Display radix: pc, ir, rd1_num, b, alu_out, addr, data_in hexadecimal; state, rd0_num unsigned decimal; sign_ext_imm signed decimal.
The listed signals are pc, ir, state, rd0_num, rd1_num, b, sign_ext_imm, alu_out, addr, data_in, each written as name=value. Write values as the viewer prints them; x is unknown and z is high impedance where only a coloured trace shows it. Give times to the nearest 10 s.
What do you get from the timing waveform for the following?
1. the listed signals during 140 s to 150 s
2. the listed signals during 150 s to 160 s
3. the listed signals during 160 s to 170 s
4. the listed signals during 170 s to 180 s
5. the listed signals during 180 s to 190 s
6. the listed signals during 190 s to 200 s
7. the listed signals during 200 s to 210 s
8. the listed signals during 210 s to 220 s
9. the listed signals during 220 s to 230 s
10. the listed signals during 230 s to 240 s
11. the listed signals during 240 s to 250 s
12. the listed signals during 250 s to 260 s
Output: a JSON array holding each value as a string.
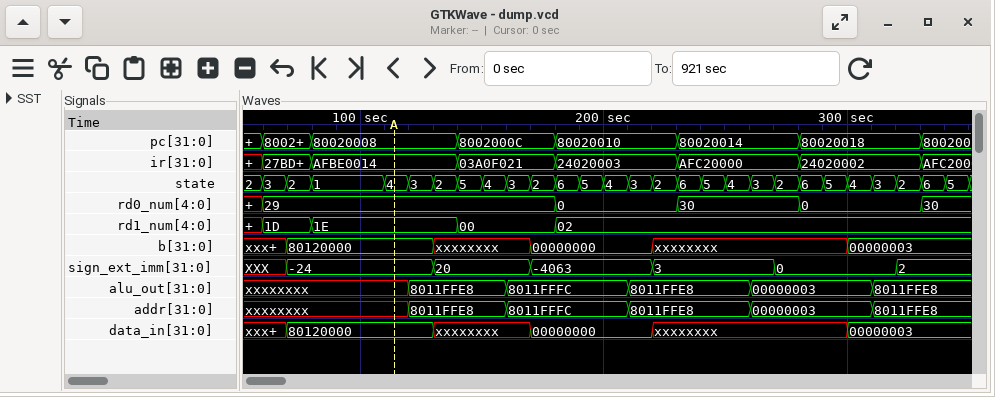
["pc=8002000C, ir=03A0F021, state=5, rd0_num=29, rd1_num=00, b=xxxxxxxx, sign_ext_imm=20, alu_out=8011FFE8, addr=8011FFE8, data_in=xxxxxxxx", "pc=8002000C, ir=03A0F021, state=4, rd0_num=29, rd1_num=00, b=xxxxxxxx, sign_ext_imm=20, alu_out=8011FFE8, addr=8011FFE8, data_in=xxxxxxxx", "pc=8002000C, ir=03A0F021, state=3, rd0_num=29, rd1_num=00, b=xxxxxxxx, sign_ext_imm=20, alu_out=8011FFFC, addr=8011FFFC, data_in=xxxxxxxx", "pc=8002000C, ir=03A0F021, state=2, rd0_num=29, rd1_num=00, b=00000000, sign_ext_imm=-4063, alu_out=8011FFFC, addr=8011FFFC, data_in=00000000", "pc=80020010, ir=24020003, state=6, rd0_num=0, rd1_num=02, b=00000000, sign_ext_imm=-4063, alu_out=8011FFFC, addr=8011FFFC, data_in=00000000", "pc=80020010, ir=24020003, state=5, rd0_num=0, rd1_num=02, b=00000000, sign_ext_imm=-4063, alu_out=8011FFFC, addr=8011FFFC, data_in=00000000", "pc=80020010, ir=24020003, state=4, rd0_num=0, rd1_num=02, b=00000000, sign_ext_imm=-4063, alu_out=8011FFFC, addr=8011FFFC, data_in=00000000", "pc=80020010, ir=24020003, state=3, rd0_num=0, rd1_num=02, b=00000000, sign_ext_imm=-4063, alu_out=8011FFE8, addr=8011FFE8, data_in=00000000", "pc=80020010, ir=24020003, state=2, rd0_num=0, rd1_num=02, b=xxxxxxxx, sign_ext_imm=3, alu_out=8011FFE8, addr=8011FFE8, data_in=xxxxxxxx", "pc=80020014, ir=AFC20000, state=6, rd0_num=30, rd1_num=02, b=xxxxxxxx, sign_ext_imm=3, alu_out=8011FFE8, addr=8011FFE8, data_in=xxxxxxxx", "pc=80020014, ir=AFC20000, state=5, rd0_num=30, rd1_num=02, b=xxxxxxxx, sign_ext_imm=3, alu_out=8011FFE8, addr=8011FFE8, data_in=xxxxxxxx", "pc=80020014, ir=AFC20000, state=4, rd0_num=30, rd1_num=02, b=xxxxxxxx, sign_ext_imm=3, alu_out=8011FFE8, addr=8011FFE8, data_in=xxxxxxxx"]
